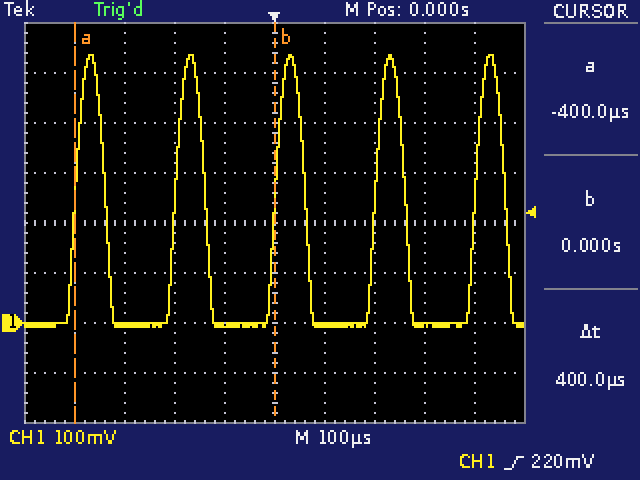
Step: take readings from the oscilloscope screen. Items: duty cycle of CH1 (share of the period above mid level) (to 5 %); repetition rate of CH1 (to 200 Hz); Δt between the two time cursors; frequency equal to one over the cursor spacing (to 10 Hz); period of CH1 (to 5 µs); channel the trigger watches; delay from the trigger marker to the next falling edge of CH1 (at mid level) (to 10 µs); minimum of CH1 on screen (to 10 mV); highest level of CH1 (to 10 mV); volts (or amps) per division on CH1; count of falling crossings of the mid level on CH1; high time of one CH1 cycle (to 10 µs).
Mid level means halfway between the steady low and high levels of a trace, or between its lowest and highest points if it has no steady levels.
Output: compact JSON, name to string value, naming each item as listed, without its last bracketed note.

{"duty cycle of CH1 (share of the period above mid level)": "30 %", "repetition rate of CH1": "5.0 kHz", "Δt between the two time cursors": "400 µs", "frequency equal to one over the cursor spacing": "2.50 kHz", "period of CH1": "200 µs", "channel the trigger watches": "CH1", "delay from the trigger marker to the next falling edge of CH1 (at mid level)": "60 µs", "minimum of CH1 on screen": "-10 mV", "highest level of CH1": "540 mV", "volts (or amps) per division on CH1": "100 mV", "count of falling crossings of the mid level on CH1": "5", "high time of one CH1 cycle": "60 µs"}
